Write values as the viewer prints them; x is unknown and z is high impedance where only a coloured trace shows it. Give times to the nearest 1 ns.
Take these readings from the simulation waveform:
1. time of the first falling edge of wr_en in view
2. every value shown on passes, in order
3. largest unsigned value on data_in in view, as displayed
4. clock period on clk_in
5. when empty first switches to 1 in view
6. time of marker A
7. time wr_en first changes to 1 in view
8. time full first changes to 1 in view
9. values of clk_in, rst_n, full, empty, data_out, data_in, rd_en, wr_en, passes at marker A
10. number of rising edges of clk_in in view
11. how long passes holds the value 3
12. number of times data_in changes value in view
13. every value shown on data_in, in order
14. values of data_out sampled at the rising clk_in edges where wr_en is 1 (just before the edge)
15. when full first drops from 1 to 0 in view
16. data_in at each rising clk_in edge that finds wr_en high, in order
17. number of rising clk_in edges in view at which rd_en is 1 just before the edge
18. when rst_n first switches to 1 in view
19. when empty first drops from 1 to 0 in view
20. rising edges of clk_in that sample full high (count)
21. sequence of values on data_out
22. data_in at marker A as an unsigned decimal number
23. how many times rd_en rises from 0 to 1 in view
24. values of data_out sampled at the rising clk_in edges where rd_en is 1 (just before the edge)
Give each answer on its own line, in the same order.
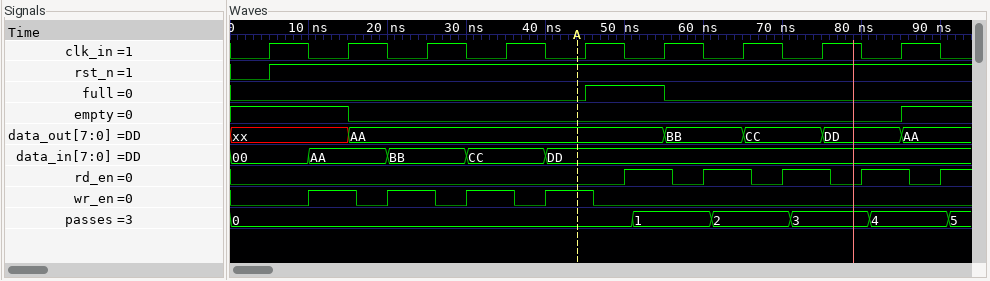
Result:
16 ns
0, 1, 2, 3, 4, 5
DD
10 ns
85 ns
44 ns
10 ns
45 ns
clk_in=0, rst_n=1, full=0, empty=0, data_out=AA, data_in=DD, rd_en=0, wr_en=1, passes=0
9
10 ns
4
00, AA, BB, CC, DD
xx, AA, AA, AA
55 ns
AA, BB, CC, DD
4
5 ns
15 ns
1
xx, AA, BB, CC, DD, AA
221
5
AA, BB, CC, DD
